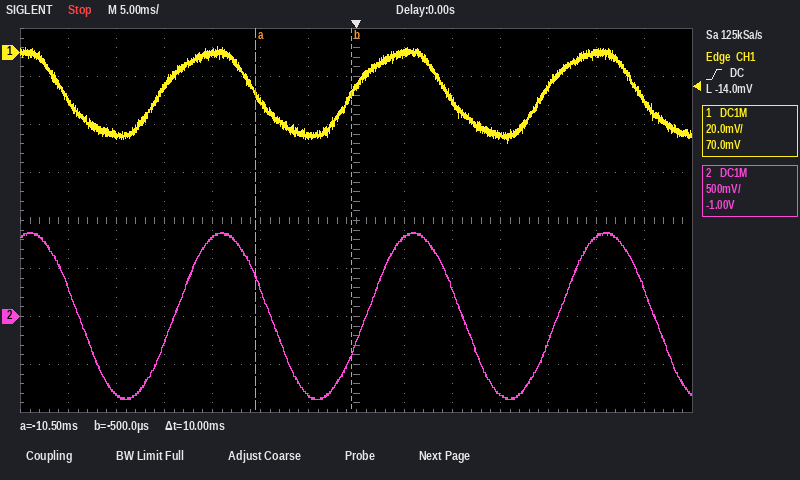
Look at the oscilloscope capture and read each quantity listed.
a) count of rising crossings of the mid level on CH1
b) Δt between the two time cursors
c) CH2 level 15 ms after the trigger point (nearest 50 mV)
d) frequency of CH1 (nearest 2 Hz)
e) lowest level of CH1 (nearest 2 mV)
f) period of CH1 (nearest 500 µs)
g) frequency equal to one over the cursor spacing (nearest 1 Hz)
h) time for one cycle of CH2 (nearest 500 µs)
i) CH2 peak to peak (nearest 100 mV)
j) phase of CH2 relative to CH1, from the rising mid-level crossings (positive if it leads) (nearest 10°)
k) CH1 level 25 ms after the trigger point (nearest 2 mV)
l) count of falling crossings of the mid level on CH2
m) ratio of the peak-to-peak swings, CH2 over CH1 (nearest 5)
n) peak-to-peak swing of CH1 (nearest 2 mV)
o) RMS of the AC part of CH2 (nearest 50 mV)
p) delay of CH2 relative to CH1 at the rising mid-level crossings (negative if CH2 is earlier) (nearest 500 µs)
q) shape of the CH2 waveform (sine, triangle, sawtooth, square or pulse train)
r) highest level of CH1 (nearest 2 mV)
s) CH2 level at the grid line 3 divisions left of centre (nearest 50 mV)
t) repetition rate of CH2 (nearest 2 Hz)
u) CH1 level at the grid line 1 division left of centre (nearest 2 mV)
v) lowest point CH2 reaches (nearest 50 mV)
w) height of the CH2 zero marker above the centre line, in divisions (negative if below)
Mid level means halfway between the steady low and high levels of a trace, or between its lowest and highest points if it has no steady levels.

3
10 ms
-800 mV
50 Hz
-38 mV
20.0 ms
100 Hz
20.0 ms
1.70 V
-30°
0 mV
4
45
40 mV
600 mV
+1.5 ms
sine
2 mV
800 mV
50 Hz
-34 mV
-850 mV
-2.0 div
